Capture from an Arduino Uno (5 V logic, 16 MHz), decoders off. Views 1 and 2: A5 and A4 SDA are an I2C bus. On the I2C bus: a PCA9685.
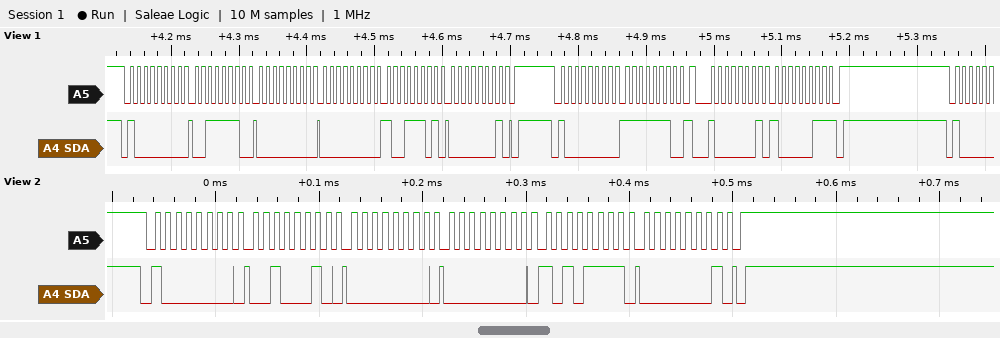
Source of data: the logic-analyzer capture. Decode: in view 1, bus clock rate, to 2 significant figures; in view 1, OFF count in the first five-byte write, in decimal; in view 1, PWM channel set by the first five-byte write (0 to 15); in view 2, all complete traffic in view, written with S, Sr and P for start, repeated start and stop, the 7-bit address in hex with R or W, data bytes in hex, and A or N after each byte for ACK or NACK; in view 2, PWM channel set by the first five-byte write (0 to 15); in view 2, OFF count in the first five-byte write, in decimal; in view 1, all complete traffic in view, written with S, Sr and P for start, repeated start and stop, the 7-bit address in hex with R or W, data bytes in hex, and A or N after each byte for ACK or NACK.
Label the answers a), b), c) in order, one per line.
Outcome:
a) 100 kHz
b) 413
c) 14
d) S 40W A 22 A 00 A 00 A AF A 01 A P
e) 7
f) 431
g) S 40W A 3E A 00 A 00 A 9D A 01 A P S 40W A FE A Sr 40R A 83 N P
